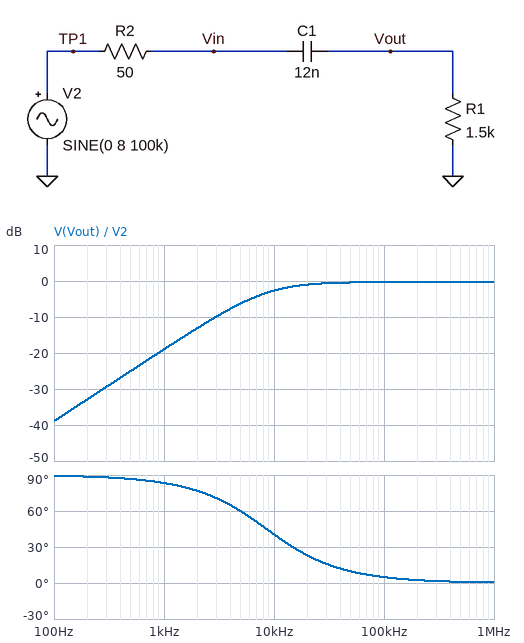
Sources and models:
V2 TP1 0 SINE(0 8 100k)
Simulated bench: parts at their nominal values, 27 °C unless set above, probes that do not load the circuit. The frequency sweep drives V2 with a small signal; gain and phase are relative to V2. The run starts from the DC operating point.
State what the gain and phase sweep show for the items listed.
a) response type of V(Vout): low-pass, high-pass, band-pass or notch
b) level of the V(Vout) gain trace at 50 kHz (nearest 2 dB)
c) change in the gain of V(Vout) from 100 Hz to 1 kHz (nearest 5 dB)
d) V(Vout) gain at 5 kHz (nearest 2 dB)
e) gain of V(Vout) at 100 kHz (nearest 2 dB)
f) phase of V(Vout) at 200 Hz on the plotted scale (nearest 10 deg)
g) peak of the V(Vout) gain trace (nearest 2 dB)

high-pass
0 dB
20 dB
-6 dB
0 dB
90 deg
0 dB
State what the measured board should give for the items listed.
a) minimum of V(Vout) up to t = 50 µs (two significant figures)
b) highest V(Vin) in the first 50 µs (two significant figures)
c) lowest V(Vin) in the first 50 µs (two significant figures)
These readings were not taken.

-8.2 V
7.8 V
-7.7 V
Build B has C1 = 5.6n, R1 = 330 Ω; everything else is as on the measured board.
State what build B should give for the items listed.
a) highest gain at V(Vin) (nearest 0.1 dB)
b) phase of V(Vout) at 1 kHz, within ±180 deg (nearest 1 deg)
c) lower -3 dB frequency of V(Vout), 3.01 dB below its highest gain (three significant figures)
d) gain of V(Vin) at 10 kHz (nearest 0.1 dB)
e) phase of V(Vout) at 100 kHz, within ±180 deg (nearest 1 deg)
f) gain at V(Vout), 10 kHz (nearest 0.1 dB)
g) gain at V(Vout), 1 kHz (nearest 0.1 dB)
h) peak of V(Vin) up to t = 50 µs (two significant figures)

0 dB
89 deg
74.8 kHz
0 dB
37 deg
-18.8 dB
-38.7 dB
7.5 V
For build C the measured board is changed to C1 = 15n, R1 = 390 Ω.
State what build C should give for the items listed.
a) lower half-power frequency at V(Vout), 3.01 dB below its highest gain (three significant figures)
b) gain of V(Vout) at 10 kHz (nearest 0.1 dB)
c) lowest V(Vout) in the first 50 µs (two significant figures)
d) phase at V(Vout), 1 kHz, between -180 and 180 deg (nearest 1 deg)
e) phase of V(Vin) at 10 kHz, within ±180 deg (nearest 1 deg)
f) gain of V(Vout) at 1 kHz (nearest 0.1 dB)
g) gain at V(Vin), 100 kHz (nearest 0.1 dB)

24.1 kHz
-9.4 dB
-7.4 V
88 deg
-2 deg
-28.7 dB
-1.0 dB
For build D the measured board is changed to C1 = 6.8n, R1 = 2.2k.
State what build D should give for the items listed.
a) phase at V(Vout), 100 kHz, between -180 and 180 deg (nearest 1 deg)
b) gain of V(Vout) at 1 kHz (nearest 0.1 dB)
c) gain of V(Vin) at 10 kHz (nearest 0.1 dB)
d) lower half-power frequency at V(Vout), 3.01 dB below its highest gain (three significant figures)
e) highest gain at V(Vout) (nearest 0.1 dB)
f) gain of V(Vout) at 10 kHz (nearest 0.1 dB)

6 deg
-20.6 dB
-0.1 dB
10.4 kHz
-0.2 dB
-3.4 dB
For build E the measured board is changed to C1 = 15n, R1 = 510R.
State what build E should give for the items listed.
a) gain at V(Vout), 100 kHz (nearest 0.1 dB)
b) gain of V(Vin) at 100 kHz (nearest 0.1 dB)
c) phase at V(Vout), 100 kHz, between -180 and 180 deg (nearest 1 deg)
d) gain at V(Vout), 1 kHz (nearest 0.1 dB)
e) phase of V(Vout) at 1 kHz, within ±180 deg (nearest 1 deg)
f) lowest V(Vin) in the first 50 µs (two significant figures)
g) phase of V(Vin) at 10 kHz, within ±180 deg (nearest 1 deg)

-1.0 dB
-0.8 dB
11 deg
-26.4 dB
87 deg
-7.3 V
-2 deg
